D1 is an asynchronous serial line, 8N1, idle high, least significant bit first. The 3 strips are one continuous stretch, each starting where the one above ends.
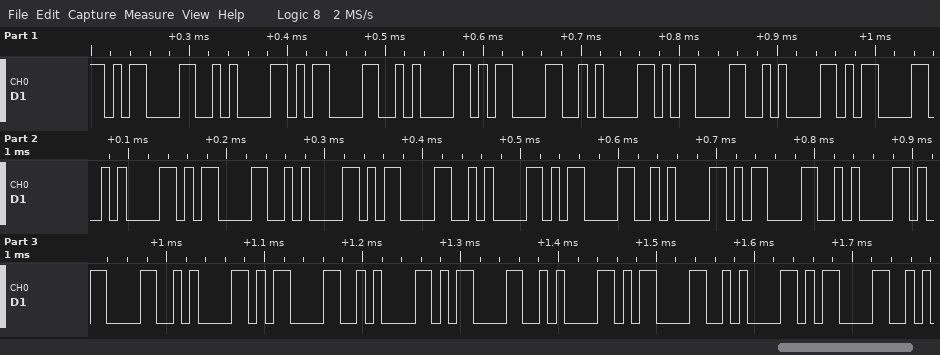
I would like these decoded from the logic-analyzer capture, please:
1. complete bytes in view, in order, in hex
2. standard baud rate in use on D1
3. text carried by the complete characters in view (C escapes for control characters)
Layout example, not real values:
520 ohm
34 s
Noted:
0D 0A 0D 0A 0D 0A 0D 0A 0D 0A 0D 0A 0D 0A 0D 0A 0D 0A 0D 0A 0D 0A 0D 0A 0D 0A 0D
115200 baud
"\r\n\r\n\r\n\r\n\r\n\r\n\r\n\r\n\r\n\r\n\r\n\r\n\r\n\r"
